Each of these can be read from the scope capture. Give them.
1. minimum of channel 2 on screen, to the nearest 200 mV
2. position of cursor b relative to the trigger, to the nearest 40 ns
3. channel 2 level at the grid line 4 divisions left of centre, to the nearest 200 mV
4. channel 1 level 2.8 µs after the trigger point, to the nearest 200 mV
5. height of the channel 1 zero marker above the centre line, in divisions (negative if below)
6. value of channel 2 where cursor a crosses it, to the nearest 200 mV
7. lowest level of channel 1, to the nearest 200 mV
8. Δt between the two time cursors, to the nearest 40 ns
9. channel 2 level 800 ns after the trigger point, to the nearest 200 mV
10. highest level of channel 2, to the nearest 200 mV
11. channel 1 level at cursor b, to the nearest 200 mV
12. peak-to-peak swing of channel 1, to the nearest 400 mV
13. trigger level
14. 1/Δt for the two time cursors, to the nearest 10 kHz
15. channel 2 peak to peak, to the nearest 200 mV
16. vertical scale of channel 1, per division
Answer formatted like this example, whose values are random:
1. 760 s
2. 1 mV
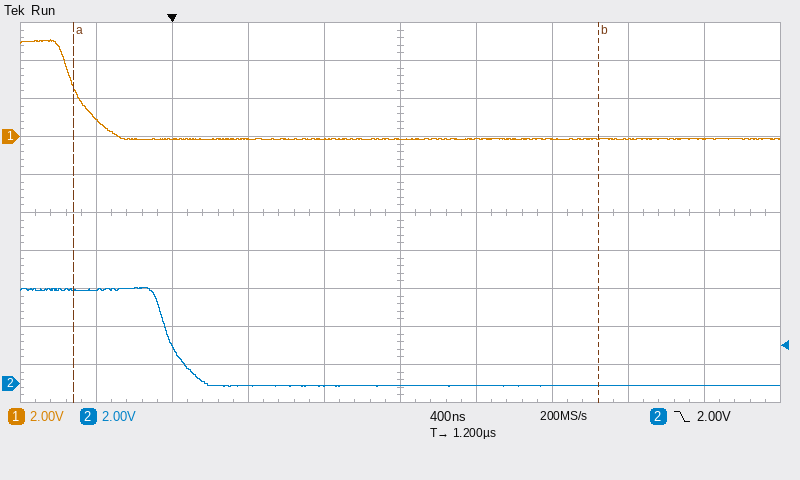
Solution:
1. -200 mV
2. +2.24 µs
3. 5.0 V
4. -200 mV
5. +2.0 div
6. 5.0 V
7. -200 mV
8. 2.76 µs
9. -200 mV
10. 5.0 V
11. -200 mV
12. 5.2 V
13. 2.00 V
14. 360 kHz
15. 5.2 V
16. 2 V
